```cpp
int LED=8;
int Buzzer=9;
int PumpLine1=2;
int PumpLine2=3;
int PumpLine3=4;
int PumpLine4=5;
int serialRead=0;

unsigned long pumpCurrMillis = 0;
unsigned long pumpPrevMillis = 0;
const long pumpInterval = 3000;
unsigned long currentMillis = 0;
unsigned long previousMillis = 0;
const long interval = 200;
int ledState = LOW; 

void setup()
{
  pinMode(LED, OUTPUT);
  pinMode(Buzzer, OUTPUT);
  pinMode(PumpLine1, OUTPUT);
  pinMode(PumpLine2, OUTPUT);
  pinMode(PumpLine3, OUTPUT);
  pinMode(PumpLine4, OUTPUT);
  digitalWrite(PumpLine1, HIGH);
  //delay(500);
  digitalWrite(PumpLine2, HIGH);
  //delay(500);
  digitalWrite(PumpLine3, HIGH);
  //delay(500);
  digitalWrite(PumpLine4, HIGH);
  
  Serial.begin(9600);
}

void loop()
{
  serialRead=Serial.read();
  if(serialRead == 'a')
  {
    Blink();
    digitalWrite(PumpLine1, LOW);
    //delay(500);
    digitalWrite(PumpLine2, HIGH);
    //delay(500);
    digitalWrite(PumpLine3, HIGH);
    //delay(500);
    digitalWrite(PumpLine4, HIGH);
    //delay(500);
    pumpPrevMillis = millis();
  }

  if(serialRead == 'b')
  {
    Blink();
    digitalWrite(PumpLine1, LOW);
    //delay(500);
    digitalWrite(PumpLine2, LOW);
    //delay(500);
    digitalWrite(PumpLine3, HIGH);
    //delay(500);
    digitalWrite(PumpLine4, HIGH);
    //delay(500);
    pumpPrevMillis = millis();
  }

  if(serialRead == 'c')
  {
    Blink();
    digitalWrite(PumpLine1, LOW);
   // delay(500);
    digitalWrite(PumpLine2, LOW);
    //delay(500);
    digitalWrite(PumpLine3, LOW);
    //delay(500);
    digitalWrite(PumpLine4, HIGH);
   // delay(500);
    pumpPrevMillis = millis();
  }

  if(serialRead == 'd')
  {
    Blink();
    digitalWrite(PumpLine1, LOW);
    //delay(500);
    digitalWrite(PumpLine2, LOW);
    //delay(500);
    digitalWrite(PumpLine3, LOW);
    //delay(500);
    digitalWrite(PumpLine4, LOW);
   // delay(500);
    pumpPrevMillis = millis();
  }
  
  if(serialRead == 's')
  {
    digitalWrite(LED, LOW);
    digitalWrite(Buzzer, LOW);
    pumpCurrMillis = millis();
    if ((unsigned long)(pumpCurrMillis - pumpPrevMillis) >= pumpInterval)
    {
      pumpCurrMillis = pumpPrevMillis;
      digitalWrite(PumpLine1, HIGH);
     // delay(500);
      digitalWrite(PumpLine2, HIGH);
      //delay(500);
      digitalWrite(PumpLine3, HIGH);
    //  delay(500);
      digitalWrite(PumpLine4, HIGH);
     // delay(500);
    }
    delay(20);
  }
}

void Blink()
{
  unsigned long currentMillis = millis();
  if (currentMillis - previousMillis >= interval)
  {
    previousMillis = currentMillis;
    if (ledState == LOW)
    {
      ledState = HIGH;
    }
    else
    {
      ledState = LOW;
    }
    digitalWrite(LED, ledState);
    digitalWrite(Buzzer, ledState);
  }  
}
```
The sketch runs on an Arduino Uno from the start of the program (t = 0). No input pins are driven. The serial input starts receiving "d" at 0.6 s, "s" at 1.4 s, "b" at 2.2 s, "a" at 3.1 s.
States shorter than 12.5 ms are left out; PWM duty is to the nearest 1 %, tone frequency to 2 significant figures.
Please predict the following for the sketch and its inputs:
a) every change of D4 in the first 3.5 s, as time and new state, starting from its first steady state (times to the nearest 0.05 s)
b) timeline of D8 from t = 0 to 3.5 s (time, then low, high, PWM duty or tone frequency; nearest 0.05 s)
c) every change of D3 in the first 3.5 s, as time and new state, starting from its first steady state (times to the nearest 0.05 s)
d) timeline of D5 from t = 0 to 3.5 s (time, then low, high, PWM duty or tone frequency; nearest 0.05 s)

0 s high; 0.6 s low; 2.2 s high
0 s low; 0.6 s high; 1.4 s low; 3.1 s high
0 s high; 0.6 s low; 3.1 s high
0 s high; 0.6 s low; 2.2 s high
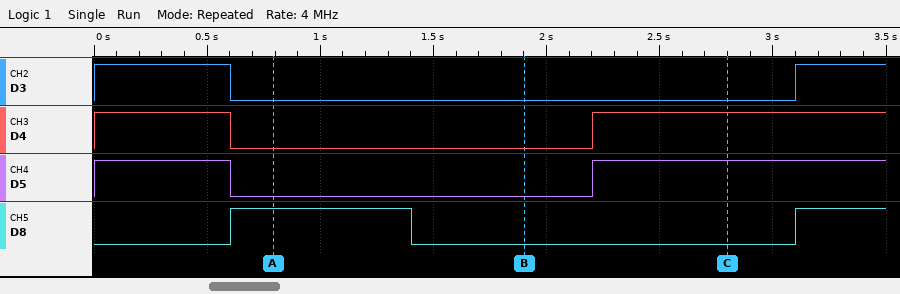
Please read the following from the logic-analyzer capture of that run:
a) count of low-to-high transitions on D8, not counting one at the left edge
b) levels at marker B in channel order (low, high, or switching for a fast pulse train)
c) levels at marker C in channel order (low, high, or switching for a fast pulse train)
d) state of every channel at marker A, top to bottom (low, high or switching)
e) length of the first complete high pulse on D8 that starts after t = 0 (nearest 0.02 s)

2
D3 low, D4 low, D5 low, D8 low
D3 low, D4 high, D5 high, D8 low
D3 low, D4 low, D5 low, D8 high
0.80 s
